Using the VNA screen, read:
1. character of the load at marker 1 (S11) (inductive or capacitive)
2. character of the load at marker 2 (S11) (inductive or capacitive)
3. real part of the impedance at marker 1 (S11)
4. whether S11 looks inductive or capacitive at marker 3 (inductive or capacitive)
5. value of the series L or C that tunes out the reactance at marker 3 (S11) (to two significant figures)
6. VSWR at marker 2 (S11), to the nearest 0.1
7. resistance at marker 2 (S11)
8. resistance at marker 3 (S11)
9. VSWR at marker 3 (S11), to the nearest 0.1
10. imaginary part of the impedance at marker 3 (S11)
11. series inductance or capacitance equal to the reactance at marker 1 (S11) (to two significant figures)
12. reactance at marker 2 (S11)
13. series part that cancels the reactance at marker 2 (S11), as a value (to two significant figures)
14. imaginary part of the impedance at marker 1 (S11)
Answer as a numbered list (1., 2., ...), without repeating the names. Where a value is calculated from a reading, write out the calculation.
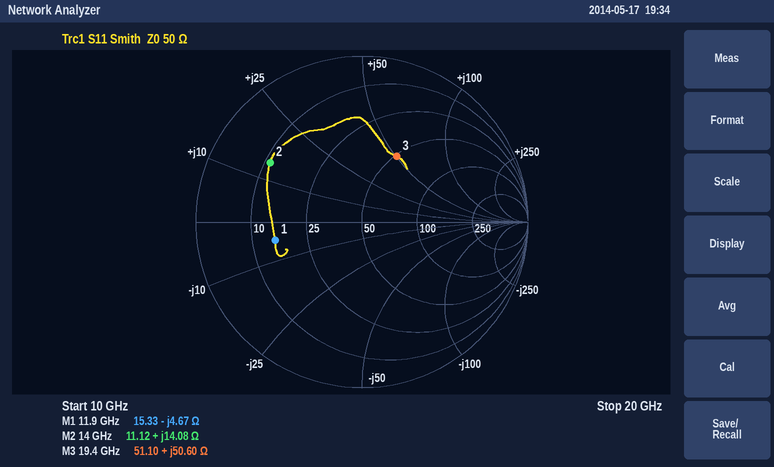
1. capacitive
2. inductive
3. 15.33 Ω
4. inductive
5. C = 1/(2π × 19.4 GHz × 50.6 Ω) ≈ 162 fF, so 160 fF to two significant figures
6. 4.9
7. 11.12 Ω
8. 51.10 Ω
9. 2.6
10. +50.60 Ω
11. C = 1/(2π × 11.9 GHz × 4.67 Ω) ≈ 2.9 pF
12. +14.08 Ω
13. C = 1/(2π × 14 GHz × 14.08 Ω) ≈ 807 fF, so 810 fF to two significant figures
14. -4.67 Ω
